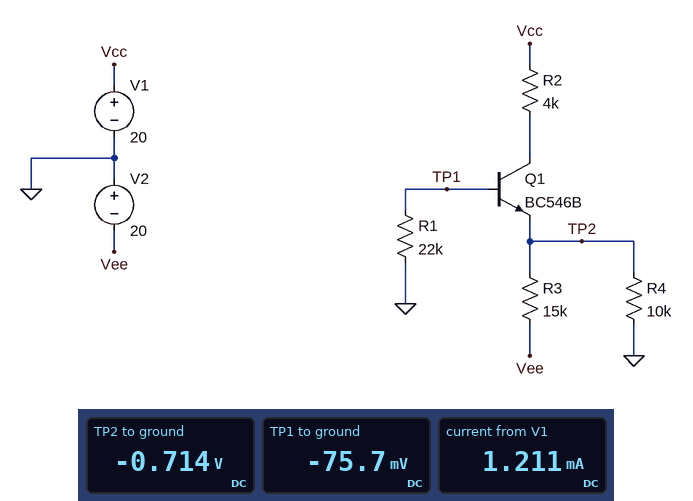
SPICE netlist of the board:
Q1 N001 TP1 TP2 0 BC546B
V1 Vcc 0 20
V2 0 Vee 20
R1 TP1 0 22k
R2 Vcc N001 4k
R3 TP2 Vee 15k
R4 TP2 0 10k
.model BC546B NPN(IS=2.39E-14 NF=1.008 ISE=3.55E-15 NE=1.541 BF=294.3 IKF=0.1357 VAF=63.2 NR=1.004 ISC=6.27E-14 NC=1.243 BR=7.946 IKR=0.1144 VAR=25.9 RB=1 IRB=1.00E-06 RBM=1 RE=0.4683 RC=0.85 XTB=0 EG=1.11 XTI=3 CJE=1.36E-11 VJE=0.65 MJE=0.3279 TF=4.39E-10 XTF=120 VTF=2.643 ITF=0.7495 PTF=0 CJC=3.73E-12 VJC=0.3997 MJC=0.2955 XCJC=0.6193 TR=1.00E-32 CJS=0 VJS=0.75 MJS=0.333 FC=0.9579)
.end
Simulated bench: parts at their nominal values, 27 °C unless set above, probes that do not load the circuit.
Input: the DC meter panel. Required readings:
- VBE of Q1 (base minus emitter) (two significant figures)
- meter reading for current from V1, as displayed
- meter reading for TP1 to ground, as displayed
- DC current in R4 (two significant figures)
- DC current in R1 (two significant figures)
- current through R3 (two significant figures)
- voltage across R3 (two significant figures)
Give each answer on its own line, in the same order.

640 mV
1.211 mA
-75.7 mV
71 µA
3.4 µA
1.3 mA
19 V
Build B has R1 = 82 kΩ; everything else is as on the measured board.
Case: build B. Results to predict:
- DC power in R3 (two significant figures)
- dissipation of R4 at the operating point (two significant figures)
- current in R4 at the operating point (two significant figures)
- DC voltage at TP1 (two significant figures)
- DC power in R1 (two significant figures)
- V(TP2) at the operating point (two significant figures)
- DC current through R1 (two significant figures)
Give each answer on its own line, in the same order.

24 mW
83 µW
91 µA
-270 mV
910 nW
-910 mV
3.3 µA
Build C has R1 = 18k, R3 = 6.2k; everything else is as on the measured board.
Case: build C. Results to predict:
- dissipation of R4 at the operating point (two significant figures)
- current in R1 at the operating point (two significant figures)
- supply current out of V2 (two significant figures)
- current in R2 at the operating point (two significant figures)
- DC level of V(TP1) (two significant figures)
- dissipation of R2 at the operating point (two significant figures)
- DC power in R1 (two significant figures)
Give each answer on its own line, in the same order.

70 µW
9.5 µA
3.1 mA
3.0 mA
-170 mV
36 mW
1.6 µW
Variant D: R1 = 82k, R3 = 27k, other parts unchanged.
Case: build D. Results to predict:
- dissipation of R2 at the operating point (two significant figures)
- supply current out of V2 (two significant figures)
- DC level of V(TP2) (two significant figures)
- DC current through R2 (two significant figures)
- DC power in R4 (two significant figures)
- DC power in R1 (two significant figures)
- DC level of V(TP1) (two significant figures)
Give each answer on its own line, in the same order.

1.6 mW
710 µA
-760 mV
630 µA
58 µW
250 nW
-140 mV
